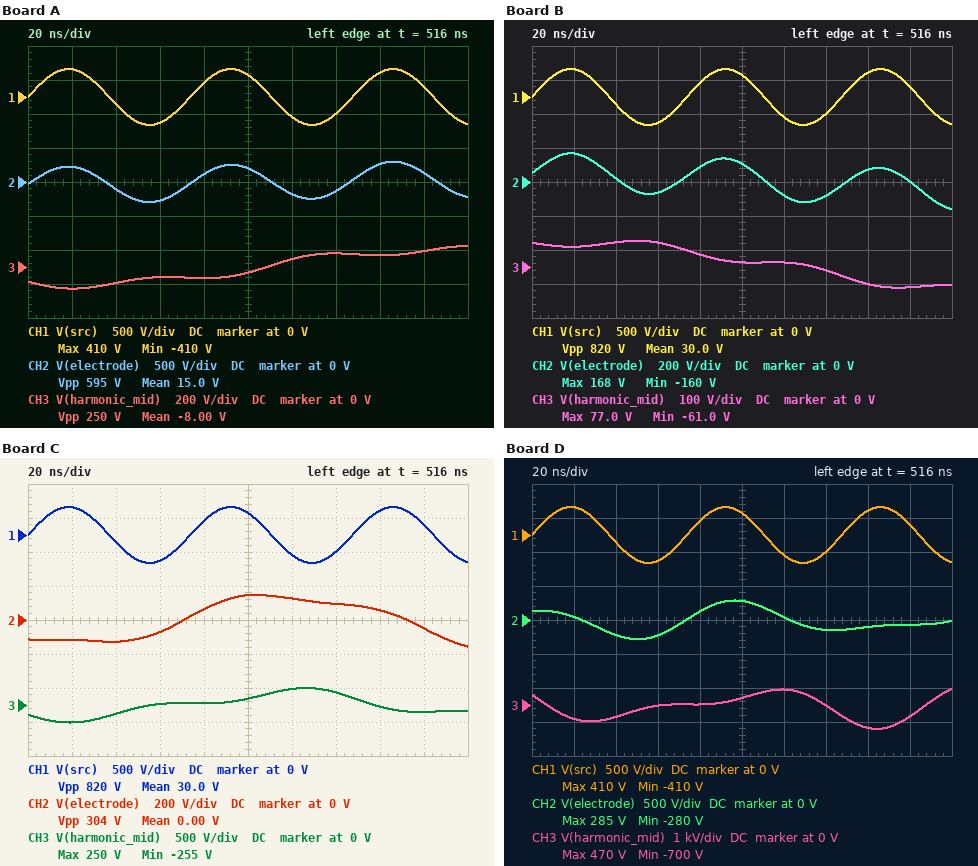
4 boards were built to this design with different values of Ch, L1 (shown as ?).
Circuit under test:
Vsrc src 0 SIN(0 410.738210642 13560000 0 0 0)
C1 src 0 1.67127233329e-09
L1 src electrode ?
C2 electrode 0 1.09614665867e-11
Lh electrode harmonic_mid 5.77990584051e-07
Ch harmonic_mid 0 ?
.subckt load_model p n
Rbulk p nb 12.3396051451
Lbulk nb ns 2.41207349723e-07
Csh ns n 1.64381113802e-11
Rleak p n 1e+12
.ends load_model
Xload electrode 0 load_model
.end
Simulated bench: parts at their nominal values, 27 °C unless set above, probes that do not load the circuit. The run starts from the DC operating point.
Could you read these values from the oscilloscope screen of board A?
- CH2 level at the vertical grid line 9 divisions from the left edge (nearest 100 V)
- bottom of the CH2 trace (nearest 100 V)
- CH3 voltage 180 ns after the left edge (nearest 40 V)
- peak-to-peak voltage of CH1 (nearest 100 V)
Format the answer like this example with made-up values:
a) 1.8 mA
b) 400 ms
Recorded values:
a) 100 V
b) -300 V
c) 80 V
d) 800 V
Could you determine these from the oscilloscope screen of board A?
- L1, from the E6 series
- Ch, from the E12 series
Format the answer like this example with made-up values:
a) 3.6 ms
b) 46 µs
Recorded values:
a) 330 nH
b) 2.7 nF
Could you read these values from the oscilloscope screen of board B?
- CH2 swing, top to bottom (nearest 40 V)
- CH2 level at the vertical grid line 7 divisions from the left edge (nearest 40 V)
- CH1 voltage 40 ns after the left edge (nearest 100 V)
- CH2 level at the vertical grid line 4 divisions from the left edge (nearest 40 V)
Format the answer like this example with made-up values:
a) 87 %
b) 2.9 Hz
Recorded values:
a) 320 V
b) -80 V
c) -100 V
d) 80 V
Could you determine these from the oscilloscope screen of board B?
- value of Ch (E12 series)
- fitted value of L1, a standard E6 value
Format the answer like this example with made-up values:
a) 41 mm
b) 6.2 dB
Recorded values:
a) 2.2 nF
b) 1.5 µH
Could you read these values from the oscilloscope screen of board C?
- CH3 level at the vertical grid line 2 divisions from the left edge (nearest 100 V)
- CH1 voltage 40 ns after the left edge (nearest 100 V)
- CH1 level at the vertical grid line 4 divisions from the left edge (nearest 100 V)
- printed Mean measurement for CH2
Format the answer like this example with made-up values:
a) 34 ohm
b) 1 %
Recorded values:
a) -100 V
b) -100 V
c) 200 V
d) 0.00 V
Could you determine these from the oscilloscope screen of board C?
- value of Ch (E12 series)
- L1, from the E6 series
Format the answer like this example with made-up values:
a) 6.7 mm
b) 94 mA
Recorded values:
a) 330 pF
b) 2.2 µH
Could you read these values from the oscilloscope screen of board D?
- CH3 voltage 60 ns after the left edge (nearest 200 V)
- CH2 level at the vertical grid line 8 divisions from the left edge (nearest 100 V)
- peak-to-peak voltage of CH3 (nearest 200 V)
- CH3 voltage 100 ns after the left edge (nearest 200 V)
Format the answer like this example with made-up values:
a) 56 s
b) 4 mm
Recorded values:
a) 0 V
b) -100 V
c) 1.2 kV
d) 200 V
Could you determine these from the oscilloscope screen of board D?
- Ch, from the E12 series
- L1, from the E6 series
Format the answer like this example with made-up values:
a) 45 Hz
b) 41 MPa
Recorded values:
a) 330 pF
b) 470 nH
